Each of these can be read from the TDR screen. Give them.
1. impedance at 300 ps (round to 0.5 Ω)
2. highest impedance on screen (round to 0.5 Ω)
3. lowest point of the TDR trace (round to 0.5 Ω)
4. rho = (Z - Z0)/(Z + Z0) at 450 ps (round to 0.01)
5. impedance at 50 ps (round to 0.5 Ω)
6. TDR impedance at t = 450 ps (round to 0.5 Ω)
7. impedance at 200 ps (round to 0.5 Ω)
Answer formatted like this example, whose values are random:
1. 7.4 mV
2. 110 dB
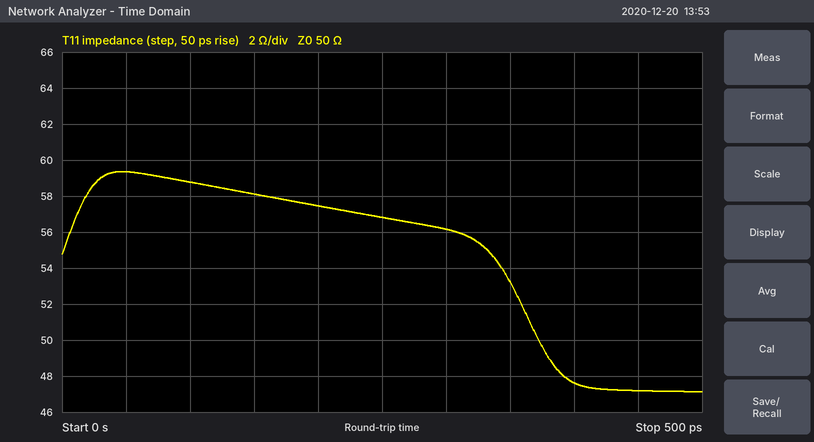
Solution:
1. 56.0 Ω
2. 59.5 Ω
3. 47.0 Ω
4. -0.03
5. 59.5 Ω
6. 47.0 Ω
7. 57.5 Ω
